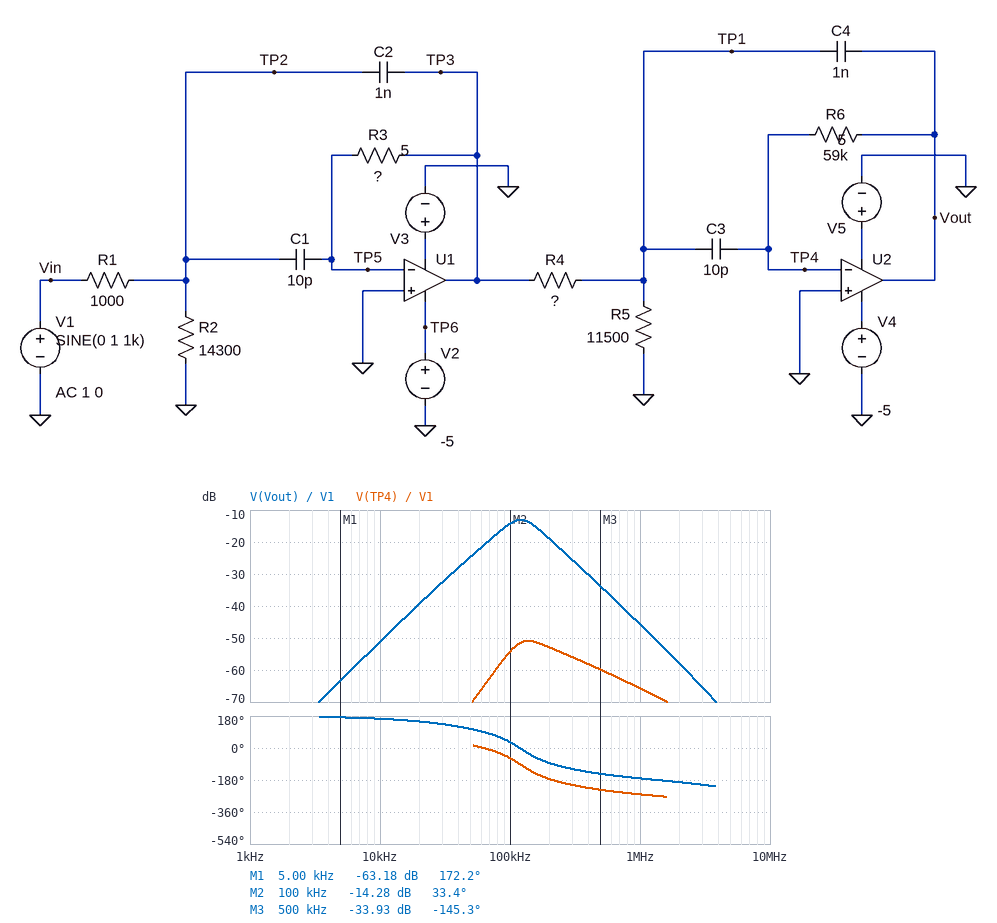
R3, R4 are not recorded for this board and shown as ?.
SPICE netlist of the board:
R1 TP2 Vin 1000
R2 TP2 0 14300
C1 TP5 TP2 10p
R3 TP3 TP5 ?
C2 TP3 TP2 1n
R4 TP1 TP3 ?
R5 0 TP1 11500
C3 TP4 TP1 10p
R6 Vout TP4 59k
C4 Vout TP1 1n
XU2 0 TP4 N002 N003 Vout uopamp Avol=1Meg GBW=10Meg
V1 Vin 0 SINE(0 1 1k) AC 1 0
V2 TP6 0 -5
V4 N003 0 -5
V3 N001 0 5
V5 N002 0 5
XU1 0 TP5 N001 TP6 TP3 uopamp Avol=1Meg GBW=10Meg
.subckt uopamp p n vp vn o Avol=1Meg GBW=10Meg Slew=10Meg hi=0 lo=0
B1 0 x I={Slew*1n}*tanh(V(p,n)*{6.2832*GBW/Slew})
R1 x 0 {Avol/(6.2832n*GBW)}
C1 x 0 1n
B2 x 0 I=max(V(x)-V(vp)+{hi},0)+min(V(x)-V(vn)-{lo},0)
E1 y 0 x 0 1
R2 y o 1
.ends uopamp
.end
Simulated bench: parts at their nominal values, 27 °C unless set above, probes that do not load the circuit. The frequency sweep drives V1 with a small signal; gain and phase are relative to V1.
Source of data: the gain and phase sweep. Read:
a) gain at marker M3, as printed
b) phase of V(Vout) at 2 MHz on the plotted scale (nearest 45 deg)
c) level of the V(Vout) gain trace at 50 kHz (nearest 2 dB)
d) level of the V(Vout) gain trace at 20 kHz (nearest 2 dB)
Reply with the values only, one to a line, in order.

-33.93 dB
-180 deg
-24 dB
-40 dB
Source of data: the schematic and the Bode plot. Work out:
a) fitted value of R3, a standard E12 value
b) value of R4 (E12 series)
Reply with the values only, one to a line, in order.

180 kΩ
4.7 kΩ
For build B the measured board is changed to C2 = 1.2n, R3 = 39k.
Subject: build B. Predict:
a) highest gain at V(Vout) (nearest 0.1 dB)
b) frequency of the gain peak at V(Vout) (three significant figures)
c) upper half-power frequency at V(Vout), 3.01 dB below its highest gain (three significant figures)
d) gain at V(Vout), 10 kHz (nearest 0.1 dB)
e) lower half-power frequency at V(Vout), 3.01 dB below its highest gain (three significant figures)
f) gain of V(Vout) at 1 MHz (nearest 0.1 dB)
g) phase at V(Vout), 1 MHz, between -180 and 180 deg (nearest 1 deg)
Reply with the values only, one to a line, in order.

-29.1 dB
185 kHz
336 kHz
-64.5 dB
95.5 kHz
-47.6 dB
-153 deg
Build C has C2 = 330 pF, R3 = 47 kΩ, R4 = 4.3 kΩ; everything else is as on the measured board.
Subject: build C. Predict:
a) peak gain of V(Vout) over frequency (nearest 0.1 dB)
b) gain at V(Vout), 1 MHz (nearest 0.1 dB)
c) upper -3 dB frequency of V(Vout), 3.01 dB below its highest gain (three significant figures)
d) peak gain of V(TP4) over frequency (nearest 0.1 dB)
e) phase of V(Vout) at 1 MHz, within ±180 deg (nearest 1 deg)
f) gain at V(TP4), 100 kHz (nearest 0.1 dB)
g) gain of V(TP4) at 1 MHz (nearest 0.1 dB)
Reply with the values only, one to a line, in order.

-18.8 dB
-34.8 dB
505 kHz
-46.9 dB
-154 deg
-68.2 dB
-54.8 dB
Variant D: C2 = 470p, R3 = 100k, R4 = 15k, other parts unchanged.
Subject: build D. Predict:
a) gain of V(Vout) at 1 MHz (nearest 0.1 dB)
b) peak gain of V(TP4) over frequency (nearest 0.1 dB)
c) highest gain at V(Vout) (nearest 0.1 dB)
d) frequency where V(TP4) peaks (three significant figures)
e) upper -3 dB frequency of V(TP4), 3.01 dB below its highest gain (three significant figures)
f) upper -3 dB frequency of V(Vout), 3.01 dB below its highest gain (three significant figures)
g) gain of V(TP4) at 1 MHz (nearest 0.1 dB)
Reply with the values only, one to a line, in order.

-49.2 dB
-56.2 dB
-23.7 dB
250 kHz
363 kHz
299 kHz
-69.2 dB
